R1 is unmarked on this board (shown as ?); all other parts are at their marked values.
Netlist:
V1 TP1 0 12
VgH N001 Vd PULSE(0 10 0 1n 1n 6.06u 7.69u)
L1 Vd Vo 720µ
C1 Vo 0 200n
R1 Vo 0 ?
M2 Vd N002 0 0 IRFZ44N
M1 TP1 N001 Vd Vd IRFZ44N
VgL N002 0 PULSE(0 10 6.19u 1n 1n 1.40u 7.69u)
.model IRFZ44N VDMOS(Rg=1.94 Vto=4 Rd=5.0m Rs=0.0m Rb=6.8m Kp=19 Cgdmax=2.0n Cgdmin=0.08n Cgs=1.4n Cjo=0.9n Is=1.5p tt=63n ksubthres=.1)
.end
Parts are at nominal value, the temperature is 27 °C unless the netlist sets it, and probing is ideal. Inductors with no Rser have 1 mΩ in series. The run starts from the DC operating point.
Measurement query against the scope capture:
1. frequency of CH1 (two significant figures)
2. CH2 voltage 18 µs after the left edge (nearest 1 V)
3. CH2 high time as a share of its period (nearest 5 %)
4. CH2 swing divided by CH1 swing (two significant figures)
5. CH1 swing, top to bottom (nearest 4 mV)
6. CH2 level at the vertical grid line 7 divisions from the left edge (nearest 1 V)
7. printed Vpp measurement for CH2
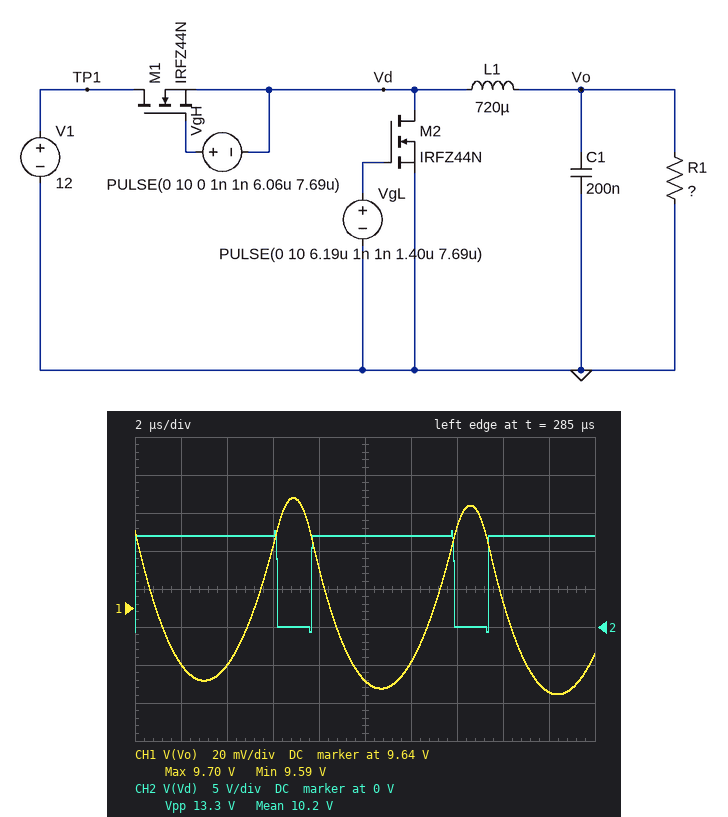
130 kHz
12 V
80 %
130
104 mV
0 V
13.3 V
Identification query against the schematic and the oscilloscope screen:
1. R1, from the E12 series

100 Ω
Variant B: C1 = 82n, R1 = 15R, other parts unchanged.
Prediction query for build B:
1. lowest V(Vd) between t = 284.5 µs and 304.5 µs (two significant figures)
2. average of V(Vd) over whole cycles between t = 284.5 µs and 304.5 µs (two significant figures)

-690 mV
9.5 V
